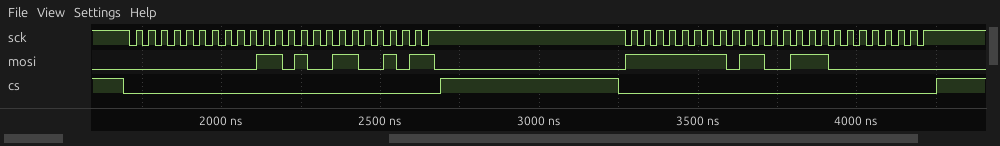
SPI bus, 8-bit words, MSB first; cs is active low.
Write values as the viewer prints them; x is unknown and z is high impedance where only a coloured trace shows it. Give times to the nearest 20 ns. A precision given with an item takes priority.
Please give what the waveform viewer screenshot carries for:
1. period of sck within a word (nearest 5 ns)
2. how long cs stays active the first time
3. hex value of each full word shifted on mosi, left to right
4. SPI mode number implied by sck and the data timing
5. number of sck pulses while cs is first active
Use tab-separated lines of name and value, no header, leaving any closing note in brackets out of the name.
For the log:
period of sck within a word	40 ns
how long cs stays active the first time	1000 ns
hex value of each full word shifted on mosi, left to right	00, 34, CB, FF, 67, 00
SPI mode number implied by sck and the data timing	3
number of sck pulses while cs is first active	24
